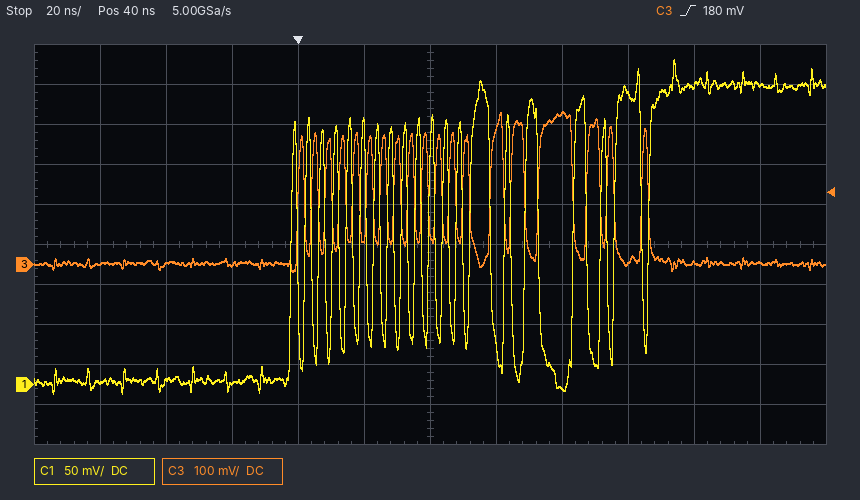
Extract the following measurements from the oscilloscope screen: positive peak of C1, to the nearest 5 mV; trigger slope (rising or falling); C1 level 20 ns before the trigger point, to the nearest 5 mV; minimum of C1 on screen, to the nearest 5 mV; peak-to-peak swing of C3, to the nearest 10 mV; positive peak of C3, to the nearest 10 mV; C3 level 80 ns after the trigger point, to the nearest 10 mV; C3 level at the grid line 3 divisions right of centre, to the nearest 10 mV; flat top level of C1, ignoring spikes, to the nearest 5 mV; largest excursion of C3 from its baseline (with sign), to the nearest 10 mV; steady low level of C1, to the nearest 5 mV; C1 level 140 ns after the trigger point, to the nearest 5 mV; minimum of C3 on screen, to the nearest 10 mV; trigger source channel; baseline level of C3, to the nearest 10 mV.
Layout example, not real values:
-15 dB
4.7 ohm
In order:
405 mV
rising
0 mV
-10 mV
400 mV
380 mV
380 mV
10 mV
375 mV
+380 mV
5 mV
375 mV
-20 mV
C3
0 mV
